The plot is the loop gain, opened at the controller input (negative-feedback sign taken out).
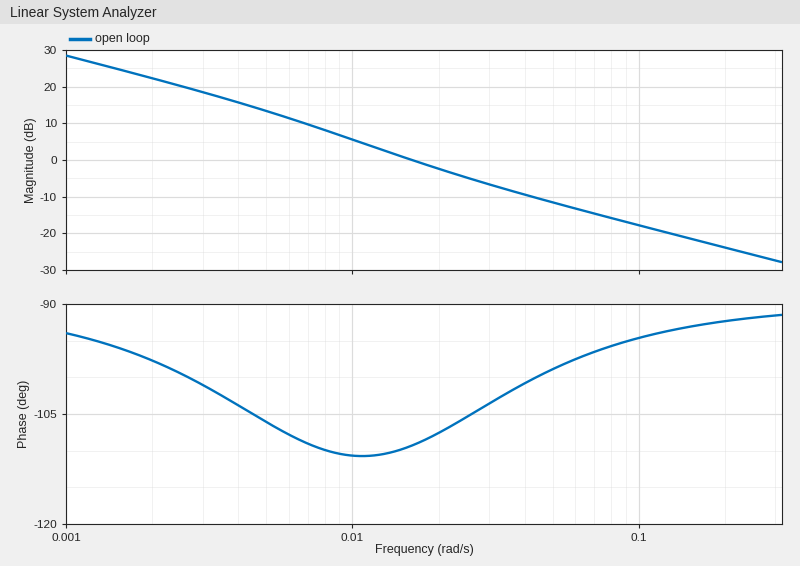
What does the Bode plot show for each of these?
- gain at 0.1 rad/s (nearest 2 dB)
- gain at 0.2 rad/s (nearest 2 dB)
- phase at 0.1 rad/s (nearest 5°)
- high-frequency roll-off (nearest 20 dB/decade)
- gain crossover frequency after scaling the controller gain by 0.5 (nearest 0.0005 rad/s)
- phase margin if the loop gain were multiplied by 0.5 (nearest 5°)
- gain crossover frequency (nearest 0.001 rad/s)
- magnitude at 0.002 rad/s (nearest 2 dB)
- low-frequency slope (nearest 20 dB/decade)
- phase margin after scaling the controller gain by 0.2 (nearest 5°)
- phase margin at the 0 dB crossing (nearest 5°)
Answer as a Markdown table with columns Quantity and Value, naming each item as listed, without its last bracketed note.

| Quantity | Value |
|---|---|
| gain at 0.1 rad/s | -18 dB |
| gain at 0.2 rad/s | -24 dB |
| phase at 0.1 rad/s | -95° |
| high-frequency roll-off | -20 dB/decade |
| gain crossover frequency after scaling the controller gain by 0.5 | 0.0095 rad/s |
| phase margin if the loop gain were multiplied by 0.5 | 70° |
| gain crossover frequency | 0.016 rad/s |
| magnitude at 0.002 rad/s | 22 dB |
| low-frequency slope | -20 dB/decade |
| phase margin after scaling the controller gain by 0.2 | 75° |
| phase margin at the 0 dB crossing | 70° |
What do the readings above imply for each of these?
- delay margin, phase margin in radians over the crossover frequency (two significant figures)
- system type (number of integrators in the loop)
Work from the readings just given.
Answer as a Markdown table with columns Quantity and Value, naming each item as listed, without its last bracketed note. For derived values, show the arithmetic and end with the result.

| Quantity | Value |
|---|---|
| delay margin, phase margin in radians over the crossover frequency | 70 × π / 180 / 0.016 = 76 s |
| system type | 1 |
